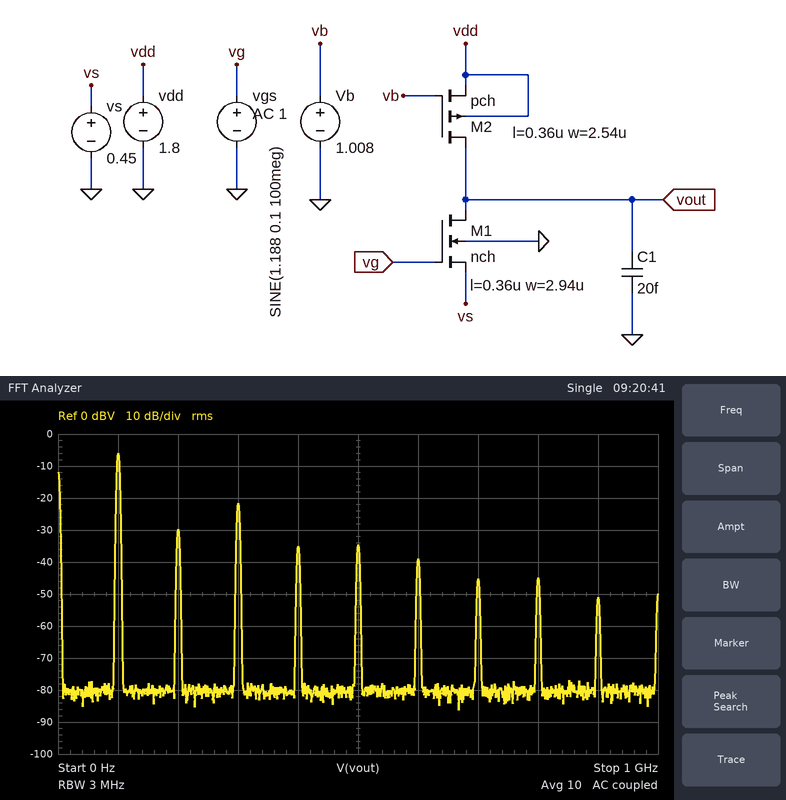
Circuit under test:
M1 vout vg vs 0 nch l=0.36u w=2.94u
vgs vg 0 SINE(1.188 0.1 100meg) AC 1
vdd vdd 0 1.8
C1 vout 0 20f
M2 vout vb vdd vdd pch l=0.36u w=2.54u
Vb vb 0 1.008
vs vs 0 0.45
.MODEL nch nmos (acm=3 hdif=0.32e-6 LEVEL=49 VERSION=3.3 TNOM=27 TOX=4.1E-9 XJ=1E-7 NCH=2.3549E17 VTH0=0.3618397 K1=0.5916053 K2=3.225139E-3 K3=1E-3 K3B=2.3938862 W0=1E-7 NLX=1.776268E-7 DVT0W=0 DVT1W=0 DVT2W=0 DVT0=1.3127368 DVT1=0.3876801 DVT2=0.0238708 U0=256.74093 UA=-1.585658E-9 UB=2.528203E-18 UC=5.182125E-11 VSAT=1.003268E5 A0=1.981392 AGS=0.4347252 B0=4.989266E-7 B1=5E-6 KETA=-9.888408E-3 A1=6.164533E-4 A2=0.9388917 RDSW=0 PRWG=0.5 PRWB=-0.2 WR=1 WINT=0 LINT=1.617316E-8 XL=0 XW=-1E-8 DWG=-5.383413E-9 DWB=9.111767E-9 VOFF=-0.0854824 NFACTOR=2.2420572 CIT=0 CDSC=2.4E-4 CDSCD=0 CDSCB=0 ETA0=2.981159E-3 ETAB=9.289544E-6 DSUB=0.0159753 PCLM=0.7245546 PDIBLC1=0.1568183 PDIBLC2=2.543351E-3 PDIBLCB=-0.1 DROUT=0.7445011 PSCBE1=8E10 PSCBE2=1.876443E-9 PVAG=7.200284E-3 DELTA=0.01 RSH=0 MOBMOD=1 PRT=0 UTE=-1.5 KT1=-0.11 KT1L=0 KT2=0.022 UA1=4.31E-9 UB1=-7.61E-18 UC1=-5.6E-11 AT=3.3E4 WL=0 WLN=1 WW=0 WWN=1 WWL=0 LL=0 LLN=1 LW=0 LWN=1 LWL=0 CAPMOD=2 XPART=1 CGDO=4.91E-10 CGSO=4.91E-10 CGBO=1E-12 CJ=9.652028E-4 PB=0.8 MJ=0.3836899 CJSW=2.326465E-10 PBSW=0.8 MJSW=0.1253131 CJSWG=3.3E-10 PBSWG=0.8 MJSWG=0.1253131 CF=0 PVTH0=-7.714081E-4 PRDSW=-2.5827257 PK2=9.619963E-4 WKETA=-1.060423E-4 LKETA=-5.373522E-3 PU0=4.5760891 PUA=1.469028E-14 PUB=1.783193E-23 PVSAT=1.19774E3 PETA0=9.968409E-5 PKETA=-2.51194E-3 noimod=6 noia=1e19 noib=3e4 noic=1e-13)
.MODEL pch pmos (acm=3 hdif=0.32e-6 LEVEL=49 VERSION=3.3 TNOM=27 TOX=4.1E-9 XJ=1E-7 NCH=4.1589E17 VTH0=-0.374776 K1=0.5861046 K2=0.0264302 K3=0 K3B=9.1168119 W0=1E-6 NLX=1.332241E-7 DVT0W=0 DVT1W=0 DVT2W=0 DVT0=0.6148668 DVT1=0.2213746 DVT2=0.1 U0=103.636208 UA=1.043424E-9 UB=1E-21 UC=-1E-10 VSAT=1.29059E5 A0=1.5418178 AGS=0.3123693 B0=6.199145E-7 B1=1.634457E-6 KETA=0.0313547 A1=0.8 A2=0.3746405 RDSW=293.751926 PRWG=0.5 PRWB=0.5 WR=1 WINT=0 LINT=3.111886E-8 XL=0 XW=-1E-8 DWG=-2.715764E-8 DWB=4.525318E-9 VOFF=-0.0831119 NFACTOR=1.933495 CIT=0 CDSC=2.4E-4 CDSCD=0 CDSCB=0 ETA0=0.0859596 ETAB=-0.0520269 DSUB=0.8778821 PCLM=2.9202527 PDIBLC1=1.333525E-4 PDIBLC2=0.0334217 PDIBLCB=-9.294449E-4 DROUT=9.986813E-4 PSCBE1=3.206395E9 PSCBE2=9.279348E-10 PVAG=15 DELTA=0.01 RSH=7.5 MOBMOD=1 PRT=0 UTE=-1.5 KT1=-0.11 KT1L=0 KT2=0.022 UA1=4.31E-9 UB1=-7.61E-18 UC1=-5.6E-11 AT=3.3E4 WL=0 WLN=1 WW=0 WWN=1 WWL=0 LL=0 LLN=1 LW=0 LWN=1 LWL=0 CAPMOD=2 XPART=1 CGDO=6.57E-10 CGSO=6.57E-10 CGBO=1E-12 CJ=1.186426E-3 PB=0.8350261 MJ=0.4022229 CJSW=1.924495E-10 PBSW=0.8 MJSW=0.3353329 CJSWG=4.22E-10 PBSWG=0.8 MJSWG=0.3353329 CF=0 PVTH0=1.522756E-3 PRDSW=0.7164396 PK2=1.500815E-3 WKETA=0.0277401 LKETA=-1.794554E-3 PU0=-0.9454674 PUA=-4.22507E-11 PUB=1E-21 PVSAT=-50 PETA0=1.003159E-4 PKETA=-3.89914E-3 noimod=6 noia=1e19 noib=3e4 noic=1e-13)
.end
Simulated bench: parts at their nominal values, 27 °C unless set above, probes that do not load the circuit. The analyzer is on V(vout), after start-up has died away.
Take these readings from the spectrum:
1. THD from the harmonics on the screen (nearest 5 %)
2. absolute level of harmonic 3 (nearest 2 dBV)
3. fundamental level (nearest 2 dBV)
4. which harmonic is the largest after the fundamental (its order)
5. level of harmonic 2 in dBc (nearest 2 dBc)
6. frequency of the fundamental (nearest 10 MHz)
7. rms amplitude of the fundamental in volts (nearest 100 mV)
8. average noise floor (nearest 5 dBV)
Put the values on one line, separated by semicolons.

20 %; -22 dBV; -6 dBV; 3; -24 dBc; 100 MHz; 500 mV; -80 dBV
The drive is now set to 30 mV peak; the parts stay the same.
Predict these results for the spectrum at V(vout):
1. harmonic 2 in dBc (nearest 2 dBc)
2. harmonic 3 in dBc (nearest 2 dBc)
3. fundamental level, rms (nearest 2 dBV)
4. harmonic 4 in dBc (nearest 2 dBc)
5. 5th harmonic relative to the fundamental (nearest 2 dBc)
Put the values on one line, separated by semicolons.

-38 dBc; -34 dBc; -10 dBV; -52 dBc; -48 dBc
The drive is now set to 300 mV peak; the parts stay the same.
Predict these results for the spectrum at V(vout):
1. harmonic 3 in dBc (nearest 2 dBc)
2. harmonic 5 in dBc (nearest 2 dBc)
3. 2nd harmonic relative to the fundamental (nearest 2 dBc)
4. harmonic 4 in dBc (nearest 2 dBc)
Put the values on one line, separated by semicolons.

-12 dBc; -22 dBc; -20 dBc; -24 dBc
